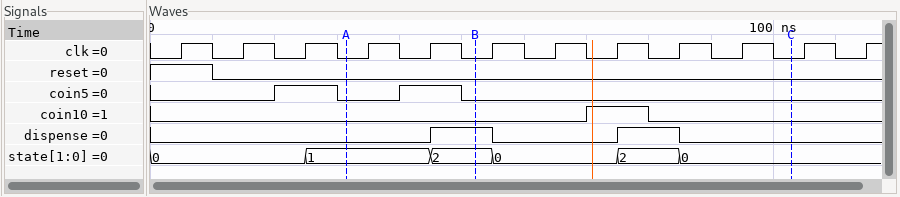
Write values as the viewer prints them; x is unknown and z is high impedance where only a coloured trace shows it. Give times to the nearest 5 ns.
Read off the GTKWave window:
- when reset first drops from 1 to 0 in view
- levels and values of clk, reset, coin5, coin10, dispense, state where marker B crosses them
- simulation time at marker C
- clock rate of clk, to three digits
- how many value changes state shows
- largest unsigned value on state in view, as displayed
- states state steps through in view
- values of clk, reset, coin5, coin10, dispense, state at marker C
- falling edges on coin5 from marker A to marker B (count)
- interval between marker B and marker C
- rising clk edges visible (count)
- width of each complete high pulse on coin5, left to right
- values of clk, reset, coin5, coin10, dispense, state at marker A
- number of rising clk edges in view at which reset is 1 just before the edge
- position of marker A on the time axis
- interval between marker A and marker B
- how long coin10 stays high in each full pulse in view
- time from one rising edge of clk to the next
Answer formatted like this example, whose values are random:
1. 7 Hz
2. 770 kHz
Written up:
1. 10 ns
2. clk=0, reset=0, coin5=0, coin10=0, dispense=1, state=2
3. 105 ns
4. 100 MHz
5. 5
6. 2
7. 0, 1, 2, 0, 2, 0
8. clk=0, reset=0, coin5=0, coin10=0, dispense=0, state=0
9. 1
10. 50 ns
11. 12
12. 10 ns, 10 ns
13. clk=0, reset=0, coin5=0, coin10=0, dispense=0, state=1
14. 1
15. 30 ns
16. 20 ns
17. 10 ns
18. 10 ns
